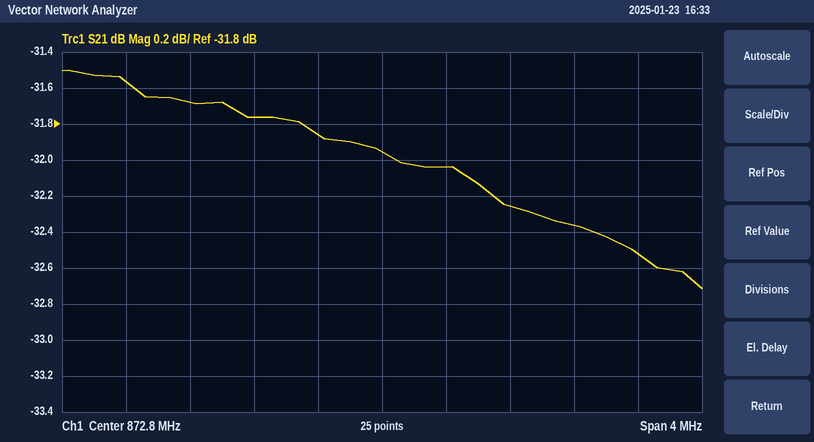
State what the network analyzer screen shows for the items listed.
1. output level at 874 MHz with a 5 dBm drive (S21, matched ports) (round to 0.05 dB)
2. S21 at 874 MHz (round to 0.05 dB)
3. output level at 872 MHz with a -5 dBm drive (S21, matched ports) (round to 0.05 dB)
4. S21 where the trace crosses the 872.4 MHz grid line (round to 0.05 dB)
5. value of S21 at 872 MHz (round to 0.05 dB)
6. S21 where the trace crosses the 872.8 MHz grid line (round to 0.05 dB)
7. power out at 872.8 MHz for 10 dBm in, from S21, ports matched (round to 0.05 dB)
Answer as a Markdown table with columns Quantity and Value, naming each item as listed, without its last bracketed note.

| Quantity | Value |
|---|---|
| output level at 874 MHz with a 5 dBm drive (S21, matched ports) | -27.35 dBm |
| S21 at 874 MHz | -32.35 dB |
| output level at 872 MHz with a -5 dBm drive (S21, matched ports) | -36.75 dBm |
| S21 where the trace crosses the 872.4 MHz grid line | -31.85 dB |
| value of S21 at 872 MHz | -31.75 dB |
| S21 where the trace crosses the 872.8 MHz grid line | -31.95 dB |
| power out at 872.8 MHz for 10 dBm in, from S21, ports matched | -21.95 dBm |
